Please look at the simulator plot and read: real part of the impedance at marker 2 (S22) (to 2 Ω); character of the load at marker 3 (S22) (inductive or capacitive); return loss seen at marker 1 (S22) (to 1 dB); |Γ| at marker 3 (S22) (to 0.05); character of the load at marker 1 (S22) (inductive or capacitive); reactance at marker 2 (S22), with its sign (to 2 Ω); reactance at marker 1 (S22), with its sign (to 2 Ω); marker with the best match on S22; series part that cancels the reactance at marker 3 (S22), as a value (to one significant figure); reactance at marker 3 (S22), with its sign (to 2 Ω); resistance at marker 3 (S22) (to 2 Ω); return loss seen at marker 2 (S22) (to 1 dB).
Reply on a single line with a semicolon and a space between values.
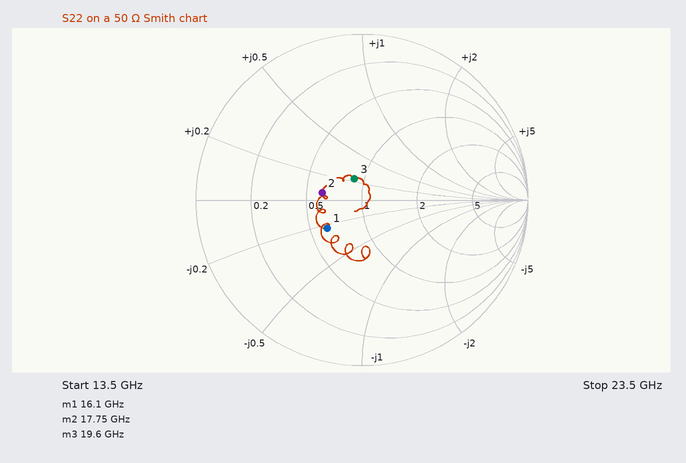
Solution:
30 Ω; inductive; 11 dB; 0.15; capacitive; +2 Ω; -12 Ω; marker 3; 700 fF; +12 Ω; 44 Ω; 12 dB
